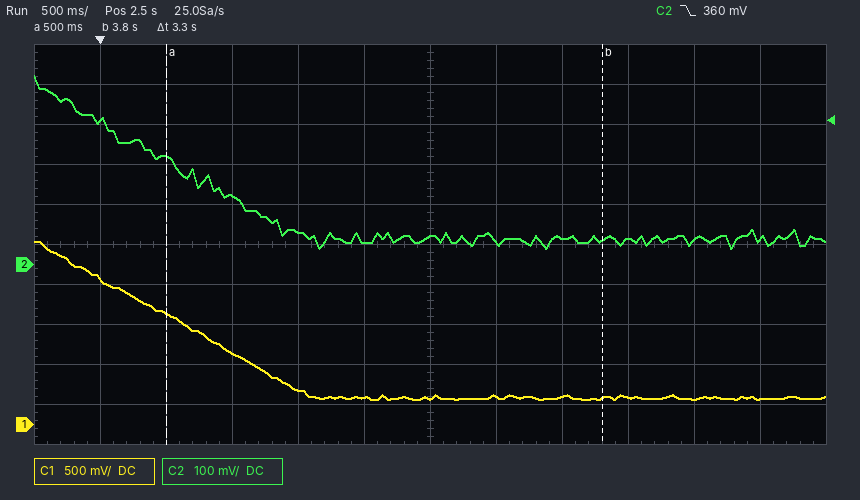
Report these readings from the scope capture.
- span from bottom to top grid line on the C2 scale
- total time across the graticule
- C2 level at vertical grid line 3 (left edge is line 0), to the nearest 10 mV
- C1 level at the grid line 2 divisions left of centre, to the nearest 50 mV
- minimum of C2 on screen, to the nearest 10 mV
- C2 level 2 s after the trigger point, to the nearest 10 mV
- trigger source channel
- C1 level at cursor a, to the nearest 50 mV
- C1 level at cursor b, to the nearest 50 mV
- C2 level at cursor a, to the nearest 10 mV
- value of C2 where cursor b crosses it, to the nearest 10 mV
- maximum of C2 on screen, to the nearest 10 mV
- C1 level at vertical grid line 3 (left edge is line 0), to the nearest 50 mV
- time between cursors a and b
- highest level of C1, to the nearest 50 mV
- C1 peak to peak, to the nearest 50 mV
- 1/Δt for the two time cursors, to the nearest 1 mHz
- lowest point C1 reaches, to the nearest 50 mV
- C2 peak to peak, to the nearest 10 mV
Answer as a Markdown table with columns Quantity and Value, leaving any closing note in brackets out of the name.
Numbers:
| Quantity | Value |
|---|---|
| span from bottom to top grid line on the C2 scale | 1 V |
| total time across the graticule | 6 s |
| C2 level at vertical grid line 3 (left edge is line 0), to the nearest 10 mV | 170 mV |
| C1 level at the grid line 2 divisions left of centre, to the nearest 50 mV | 450 mV |
| minimum of C2 on screen, to the nearest 10 mV | 40 mV |
| C2 level 2 s after the trigger point, to the nearest 10 mV | 60 mV |
| trigger source channel | C2 |
| C1 level at cursor a, to the nearest 50 mV | 1.40 V |
| C1 level at cursor b, to the nearest 50 mV | 350 mV |
| C2 level at cursor a, to the nearest 10 mV | 270 mV |
| value of C2 where cursor b crosses it, to the nearest 10 mV | 60 mV |
| maximum of C2 on screen, to the nearest 10 mV | 470 mV |
| C1 level at vertical grid line 3 (left edge is line 0), to the nearest 50 mV | 900 mV |
| time between cursors a and b | 3.3 s |
| highest level of C1, to the nearest 50 mV | 2.30 V |
| C1 peak to peak, to the nearest 50 mV | 2.00 V |
| 1/Δt for the two time cursors, to the nearest 1 mHz | 303 mHz |
| lowest point C1 reaches, to the nearest 50 mV | 300 mV |
| C2 peak to peak, to the nearest 10 mV | 430 mV |
